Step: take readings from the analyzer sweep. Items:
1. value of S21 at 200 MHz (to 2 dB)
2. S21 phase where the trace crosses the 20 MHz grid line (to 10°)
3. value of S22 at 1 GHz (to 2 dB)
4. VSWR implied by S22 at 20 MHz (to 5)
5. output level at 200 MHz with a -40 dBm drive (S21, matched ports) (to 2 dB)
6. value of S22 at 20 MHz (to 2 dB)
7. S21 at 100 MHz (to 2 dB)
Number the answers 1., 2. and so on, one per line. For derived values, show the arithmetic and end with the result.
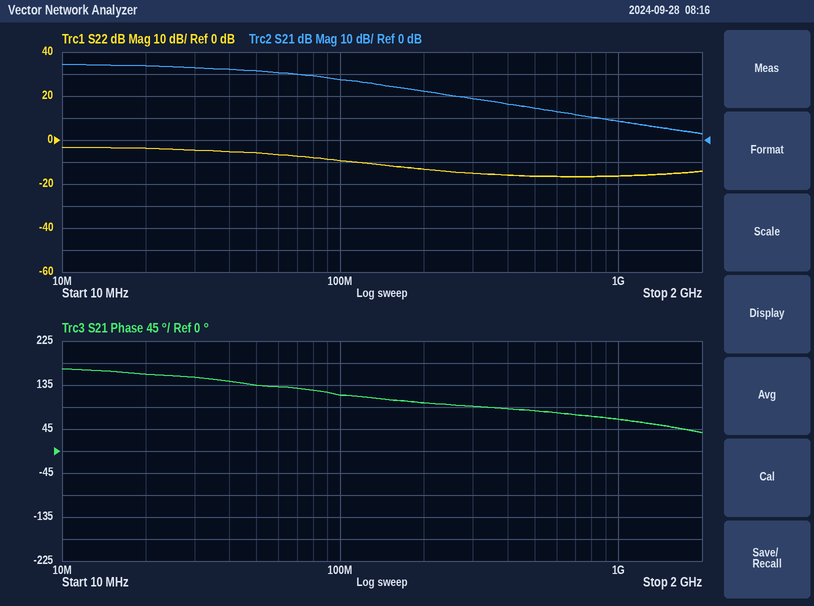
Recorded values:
1. 22 dB
2. 160°
3. -16 dB
4. |Γ| = 10^(-4/20) = 0.6310; VSWR = (1 + 0.6310)/(1 − 0.6310) ≈ 4.42, so 5 to the nearest 5
5. -40 dBm + (22 dB) = -18 dBm
6. -4 dB
7. 28 dB
